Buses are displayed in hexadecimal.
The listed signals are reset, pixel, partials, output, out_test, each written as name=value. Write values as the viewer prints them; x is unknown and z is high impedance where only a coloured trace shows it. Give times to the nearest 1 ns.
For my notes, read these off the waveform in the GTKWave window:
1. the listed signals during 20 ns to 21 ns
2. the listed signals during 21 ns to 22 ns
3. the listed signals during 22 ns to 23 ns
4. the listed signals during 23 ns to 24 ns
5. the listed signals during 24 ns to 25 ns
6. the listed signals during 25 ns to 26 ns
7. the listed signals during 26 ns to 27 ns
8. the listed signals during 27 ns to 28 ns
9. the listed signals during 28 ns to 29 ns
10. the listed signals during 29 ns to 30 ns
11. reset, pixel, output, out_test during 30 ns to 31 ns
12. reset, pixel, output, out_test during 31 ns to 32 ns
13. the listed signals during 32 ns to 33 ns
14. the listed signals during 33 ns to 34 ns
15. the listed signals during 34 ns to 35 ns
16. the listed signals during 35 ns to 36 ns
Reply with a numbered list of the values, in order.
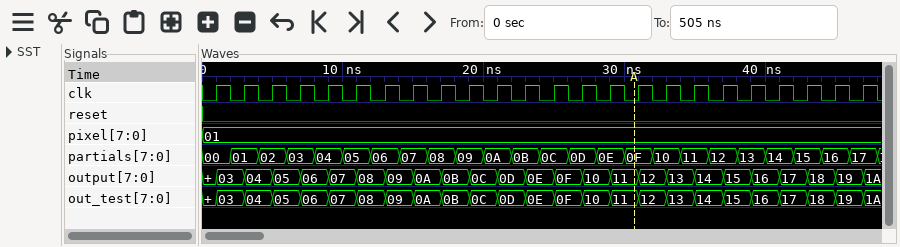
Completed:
1. reset=0, pixel=01, partials=0A, output=0C, out_test=0C
2. reset=0, pixel=01, partials=0A, output=0D, out_test=0D
3. reset=0, pixel=01, partials=0B, output=0D, out_test=0D
4. reset=0, pixel=01, partials=0B, output=0E, out_test=0E
5. reset=0, pixel=01, partials=0C, output=0E, out_test=0E
6. reset=0, pixel=01, partials=0C, output=0F, out_test=0F
7. reset=0, pixel=01, partials=0D, output=0F, out_test=0F
8. reset=0, pixel=01, partials=0D, output=10, out_test=10
9. reset=0, pixel=01, partials=0E, output=10, out_test=10
10. reset=0, pixel=01, partials=0E, output=11, out_test=11
11. reset=0, pixel=01, output=11, out_test=11
12. reset=0, pixel=01, output=12, out_test=12
13. reset=0, pixel=01, partials=10, output=12, out_test=12
14. reset=0, pixel=01, partials=10, output=13, out_test=13
15. reset=0, pixel=01, partials=11, output=13, out_test=13
16. reset=0, pixel=01, partials=11, output=14, out_test=14
